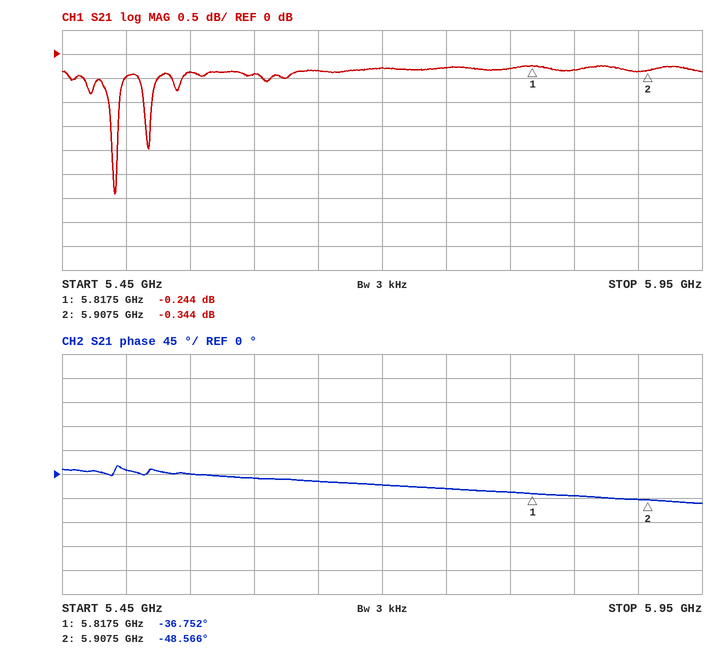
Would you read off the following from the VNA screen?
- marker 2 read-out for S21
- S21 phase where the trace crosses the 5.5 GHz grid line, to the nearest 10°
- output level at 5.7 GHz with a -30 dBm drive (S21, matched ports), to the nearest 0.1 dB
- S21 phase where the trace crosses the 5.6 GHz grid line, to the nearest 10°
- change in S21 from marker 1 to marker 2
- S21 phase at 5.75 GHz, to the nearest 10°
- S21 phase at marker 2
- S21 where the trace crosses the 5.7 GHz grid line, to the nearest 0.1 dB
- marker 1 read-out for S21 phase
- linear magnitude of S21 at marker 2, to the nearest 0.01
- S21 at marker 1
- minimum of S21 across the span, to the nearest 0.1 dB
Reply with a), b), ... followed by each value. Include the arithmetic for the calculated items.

a) -0.344 dB
b) 10°
c) -30 dBm + (-0.3 dB) = -30.3 dBm
d) -10°
e) -0.344 − (-0.244) = -0.100 dB
f) -30°
g) -48.566°
h) -0.3 dB
i) -36.752°
j) 10^(-0.344/20) ≈ 0.96
k) -0.244 dB
l) -2.9 dB
